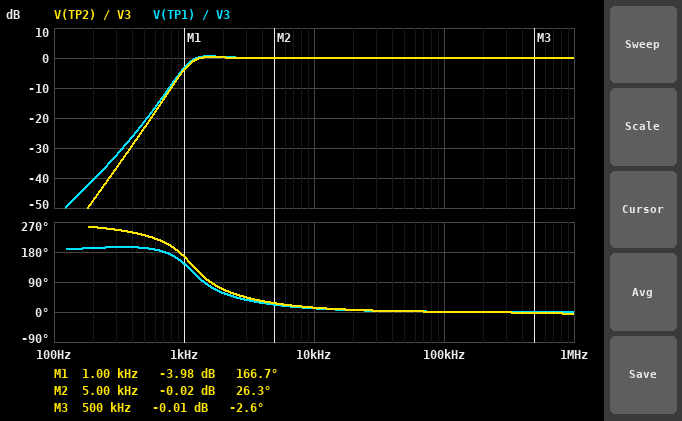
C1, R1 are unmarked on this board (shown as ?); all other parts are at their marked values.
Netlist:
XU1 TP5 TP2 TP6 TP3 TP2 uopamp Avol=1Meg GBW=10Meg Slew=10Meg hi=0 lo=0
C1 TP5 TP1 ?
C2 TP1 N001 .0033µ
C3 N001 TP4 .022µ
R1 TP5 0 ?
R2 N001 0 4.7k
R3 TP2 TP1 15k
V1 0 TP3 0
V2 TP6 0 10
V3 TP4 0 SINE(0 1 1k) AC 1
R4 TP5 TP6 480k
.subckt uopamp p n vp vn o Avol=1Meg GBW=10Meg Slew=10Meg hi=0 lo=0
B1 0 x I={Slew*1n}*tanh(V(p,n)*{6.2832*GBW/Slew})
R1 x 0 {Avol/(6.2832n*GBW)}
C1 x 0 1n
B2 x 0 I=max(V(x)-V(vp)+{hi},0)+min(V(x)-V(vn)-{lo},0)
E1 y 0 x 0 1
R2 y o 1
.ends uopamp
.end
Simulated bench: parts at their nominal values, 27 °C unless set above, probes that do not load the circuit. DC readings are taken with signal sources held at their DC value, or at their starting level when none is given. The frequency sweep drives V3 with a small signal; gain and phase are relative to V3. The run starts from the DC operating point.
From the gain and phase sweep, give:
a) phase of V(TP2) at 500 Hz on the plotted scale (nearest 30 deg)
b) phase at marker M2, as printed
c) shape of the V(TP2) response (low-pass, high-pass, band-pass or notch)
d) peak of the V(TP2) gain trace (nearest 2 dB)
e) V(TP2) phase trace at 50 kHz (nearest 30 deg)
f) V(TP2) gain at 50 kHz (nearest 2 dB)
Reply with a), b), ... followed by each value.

a) 240 deg
b) 26.3 deg
c) high-pass
d) 0 dB
e) 0 deg
f) 0 dB
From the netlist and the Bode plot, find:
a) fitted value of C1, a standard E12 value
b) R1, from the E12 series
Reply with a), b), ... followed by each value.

a) 2.7 nF
b) 220 kΩ
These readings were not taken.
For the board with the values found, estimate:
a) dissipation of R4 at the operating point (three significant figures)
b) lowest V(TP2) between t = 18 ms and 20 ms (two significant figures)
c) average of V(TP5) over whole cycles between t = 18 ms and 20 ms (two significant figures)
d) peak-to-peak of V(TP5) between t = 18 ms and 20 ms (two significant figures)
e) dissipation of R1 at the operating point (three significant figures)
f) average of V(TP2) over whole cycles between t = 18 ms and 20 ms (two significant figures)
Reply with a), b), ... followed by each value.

a) 98.0 µW
b) 2.5 V
c) 3.1 V
d) 1.3 V
e) 44.9 µW
f) 3.1 V
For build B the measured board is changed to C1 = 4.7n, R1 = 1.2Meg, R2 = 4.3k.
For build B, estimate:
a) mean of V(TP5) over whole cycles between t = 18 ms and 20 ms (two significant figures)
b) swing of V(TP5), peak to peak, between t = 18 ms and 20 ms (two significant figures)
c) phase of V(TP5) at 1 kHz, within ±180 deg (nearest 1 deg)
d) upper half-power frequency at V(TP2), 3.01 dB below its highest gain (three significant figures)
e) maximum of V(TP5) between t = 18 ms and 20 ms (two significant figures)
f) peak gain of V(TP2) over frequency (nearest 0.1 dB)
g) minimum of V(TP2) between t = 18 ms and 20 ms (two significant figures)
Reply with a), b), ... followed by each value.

a) 7.1 V
b) 1.4 V
c) 81 deg
d) 10.0 MHz
e) 7.8 V
f) 0 dB
g) 6.4 V
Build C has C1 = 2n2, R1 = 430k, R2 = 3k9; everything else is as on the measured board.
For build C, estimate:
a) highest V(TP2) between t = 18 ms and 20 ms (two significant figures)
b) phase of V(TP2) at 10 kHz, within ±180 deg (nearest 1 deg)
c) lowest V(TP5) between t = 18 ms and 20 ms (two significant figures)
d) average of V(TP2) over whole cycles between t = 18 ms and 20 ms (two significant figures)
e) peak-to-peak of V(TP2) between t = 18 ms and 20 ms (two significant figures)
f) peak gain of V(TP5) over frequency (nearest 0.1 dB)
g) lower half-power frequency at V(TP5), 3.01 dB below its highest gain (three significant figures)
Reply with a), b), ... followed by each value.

a) 5.5 V
b) 14 deg
c) 3.9 V
d) 4.7 V
e) 1.6 V
f) 0 dB
g) 956 Hz
